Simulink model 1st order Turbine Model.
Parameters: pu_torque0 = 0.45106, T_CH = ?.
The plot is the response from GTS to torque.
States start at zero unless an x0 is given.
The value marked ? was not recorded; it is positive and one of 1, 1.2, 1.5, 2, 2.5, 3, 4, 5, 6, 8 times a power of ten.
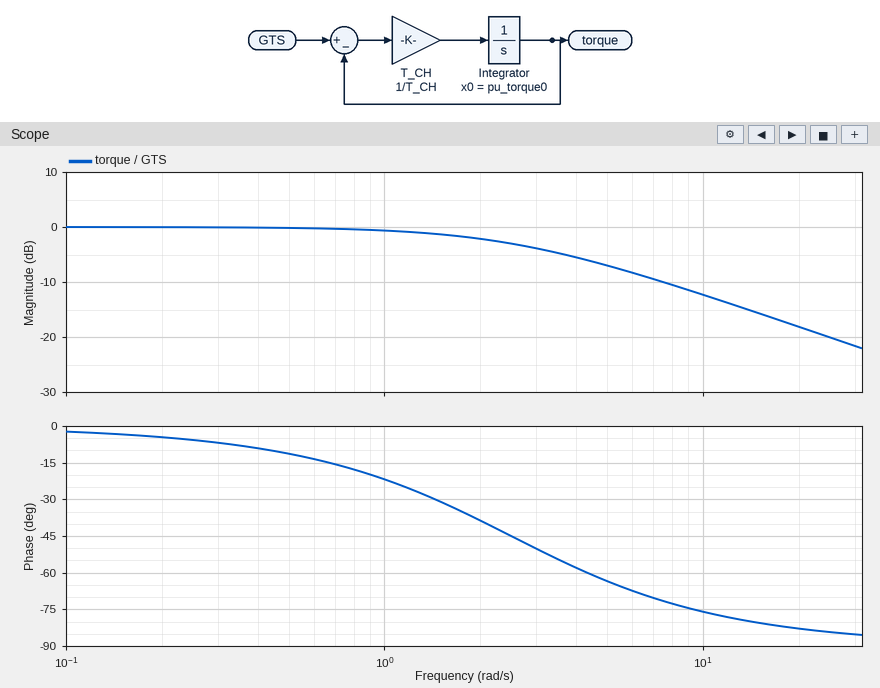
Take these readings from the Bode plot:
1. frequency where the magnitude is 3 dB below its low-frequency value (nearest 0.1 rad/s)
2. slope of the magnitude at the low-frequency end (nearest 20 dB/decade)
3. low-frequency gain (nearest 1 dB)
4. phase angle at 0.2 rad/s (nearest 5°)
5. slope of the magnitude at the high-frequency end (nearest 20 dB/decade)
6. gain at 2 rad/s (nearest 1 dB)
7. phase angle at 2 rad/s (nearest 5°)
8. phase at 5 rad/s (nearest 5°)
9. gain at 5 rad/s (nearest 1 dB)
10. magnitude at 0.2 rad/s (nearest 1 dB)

2.5 rad/s
0 dB/decade
0 dB
-5°
-20 dB/decade
-2 dB
-40°
-65°
-7 dB
0 dB
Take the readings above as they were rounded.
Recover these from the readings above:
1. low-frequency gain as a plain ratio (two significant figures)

1.0
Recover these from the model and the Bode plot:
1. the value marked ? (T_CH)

0.4
